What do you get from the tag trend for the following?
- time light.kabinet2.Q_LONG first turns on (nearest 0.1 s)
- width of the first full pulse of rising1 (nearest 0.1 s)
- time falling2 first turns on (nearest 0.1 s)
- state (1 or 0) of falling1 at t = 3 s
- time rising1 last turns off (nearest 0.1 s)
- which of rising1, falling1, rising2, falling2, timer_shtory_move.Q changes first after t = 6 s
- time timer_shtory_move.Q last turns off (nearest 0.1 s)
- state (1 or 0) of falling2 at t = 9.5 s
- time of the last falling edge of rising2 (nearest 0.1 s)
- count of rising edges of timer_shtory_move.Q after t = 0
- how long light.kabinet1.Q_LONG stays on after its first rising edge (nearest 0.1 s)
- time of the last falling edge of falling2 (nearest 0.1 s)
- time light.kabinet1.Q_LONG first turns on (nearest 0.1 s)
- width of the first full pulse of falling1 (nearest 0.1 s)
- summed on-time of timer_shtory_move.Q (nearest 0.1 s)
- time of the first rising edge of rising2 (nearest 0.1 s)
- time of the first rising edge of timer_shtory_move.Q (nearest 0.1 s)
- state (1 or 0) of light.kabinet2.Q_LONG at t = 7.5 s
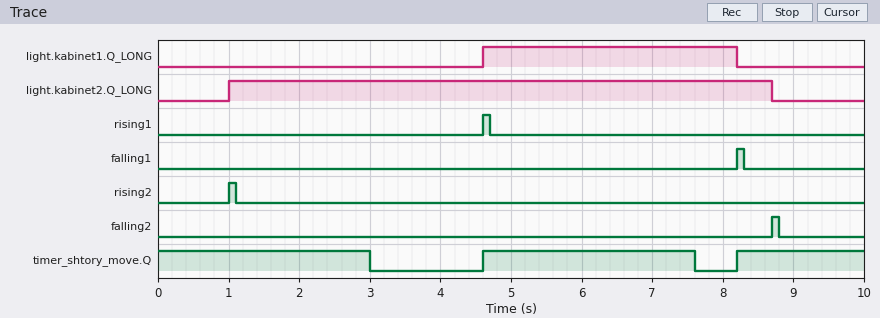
1.0 s
0.1 s
8.7 s
0
4.7 s
timer_shtory_move.Q
7.6 s
0
1.1 s
2
3.6 s
8.8 s
4.6 s
0.1 s
7.8 s
1.0 s
4.6 s
1
